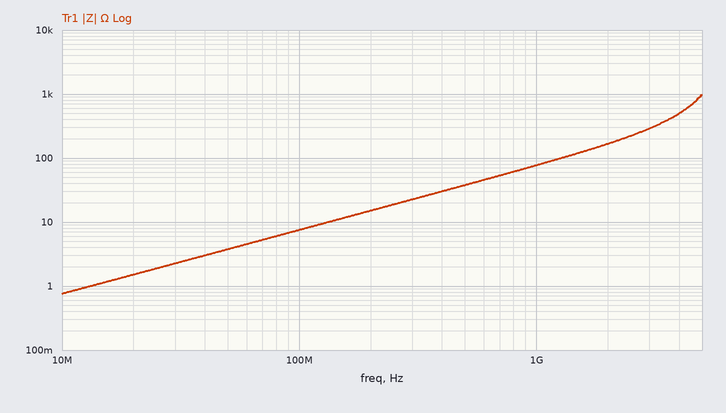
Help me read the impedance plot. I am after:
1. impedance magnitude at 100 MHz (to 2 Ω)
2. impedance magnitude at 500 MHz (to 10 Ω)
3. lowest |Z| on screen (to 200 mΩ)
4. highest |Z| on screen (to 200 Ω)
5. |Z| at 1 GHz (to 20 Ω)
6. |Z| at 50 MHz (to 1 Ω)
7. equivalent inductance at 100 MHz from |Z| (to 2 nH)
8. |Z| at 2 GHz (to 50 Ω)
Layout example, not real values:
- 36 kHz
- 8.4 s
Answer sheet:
- 8 Ω
- 40 Ω
- 800 mΩ
- 1.0 kΩ
- 80 Ω
- 4 Ω
- 12 nH
- 150 Ω
